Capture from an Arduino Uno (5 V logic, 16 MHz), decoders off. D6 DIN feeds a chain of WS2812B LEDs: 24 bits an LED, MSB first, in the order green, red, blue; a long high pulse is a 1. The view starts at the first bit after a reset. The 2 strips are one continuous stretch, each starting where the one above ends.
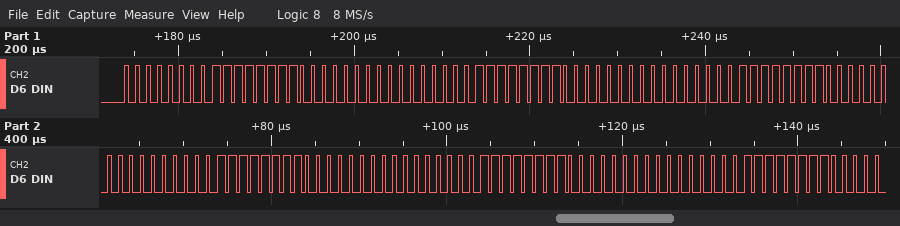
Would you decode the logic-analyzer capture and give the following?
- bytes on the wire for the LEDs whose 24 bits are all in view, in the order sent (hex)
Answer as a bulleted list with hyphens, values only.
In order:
- 00 FF 00 00 FF 00 00 FF 00 00 FF 00 00 FF 00
